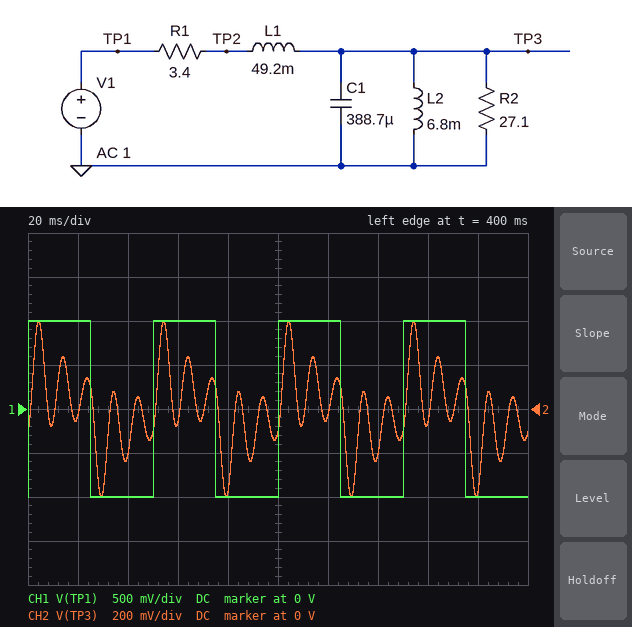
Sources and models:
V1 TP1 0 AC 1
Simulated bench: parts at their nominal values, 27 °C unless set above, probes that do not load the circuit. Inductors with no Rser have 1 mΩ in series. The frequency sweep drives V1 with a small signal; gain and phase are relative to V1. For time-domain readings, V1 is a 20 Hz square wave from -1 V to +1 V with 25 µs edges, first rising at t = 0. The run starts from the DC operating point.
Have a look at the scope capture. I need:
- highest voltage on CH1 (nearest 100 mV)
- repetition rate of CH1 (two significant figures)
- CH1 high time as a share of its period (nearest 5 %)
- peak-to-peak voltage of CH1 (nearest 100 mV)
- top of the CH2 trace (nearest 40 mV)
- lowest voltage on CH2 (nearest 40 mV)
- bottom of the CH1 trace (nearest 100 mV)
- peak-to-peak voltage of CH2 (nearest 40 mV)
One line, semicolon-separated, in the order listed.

1.0 V; 20 Hz; 50 %; 2.0 V; 400 mV; -400 mV; -1.0 V; 800 mV
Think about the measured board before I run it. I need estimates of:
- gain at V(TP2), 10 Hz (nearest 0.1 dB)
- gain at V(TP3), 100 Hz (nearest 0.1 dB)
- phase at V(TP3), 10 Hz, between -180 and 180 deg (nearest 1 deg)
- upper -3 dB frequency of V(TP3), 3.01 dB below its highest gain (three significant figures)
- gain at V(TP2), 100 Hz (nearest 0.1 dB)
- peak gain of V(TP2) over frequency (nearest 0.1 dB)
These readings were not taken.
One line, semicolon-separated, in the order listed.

-2.9 dB; -3.1 dB; 43 deg; 112 Hz; -0.6 dB; 0 dB
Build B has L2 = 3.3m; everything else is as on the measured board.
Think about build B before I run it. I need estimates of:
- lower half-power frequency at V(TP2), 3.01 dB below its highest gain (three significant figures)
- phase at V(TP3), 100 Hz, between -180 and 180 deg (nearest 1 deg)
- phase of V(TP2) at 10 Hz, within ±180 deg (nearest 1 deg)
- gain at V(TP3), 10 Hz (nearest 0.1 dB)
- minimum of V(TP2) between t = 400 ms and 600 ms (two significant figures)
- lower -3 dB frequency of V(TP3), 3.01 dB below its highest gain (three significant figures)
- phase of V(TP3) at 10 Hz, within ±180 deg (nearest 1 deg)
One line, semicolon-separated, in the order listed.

10.3 Hz; -2 deg; 46 deg; -27.1 dB; -1.7 V; 137 Hz; 45 deg
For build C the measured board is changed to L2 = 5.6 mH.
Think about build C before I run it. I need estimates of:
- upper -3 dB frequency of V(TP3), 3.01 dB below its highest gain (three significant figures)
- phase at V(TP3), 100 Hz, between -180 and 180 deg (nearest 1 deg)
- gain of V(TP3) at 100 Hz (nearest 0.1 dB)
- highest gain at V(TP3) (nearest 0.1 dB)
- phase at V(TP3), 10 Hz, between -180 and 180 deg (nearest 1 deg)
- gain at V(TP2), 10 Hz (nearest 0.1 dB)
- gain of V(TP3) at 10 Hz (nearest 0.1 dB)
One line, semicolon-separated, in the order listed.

121 Hz; -23 deg; -8.2 dB; -2.9 dB; 44 deg; -3.0 dB; -22.7 dB
